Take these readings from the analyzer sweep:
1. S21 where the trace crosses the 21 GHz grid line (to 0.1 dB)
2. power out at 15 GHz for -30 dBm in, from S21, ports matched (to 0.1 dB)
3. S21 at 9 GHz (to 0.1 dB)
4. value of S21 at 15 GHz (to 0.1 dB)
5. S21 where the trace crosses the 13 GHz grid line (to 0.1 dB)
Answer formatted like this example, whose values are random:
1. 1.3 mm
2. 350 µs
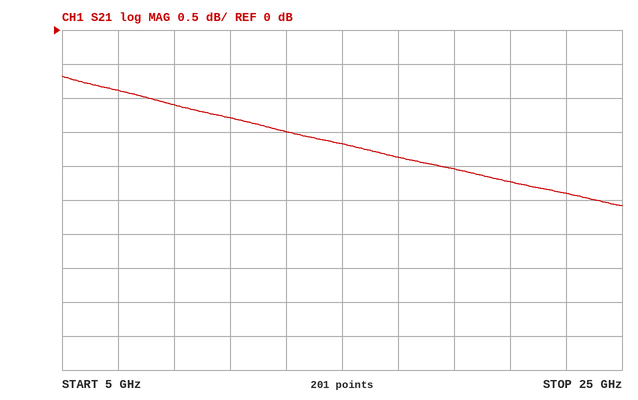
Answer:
1. -2.2 dB
2. -31.7 dBm
3. -1.1 dB
4. -1.7 dB
5. -1.5 dB
